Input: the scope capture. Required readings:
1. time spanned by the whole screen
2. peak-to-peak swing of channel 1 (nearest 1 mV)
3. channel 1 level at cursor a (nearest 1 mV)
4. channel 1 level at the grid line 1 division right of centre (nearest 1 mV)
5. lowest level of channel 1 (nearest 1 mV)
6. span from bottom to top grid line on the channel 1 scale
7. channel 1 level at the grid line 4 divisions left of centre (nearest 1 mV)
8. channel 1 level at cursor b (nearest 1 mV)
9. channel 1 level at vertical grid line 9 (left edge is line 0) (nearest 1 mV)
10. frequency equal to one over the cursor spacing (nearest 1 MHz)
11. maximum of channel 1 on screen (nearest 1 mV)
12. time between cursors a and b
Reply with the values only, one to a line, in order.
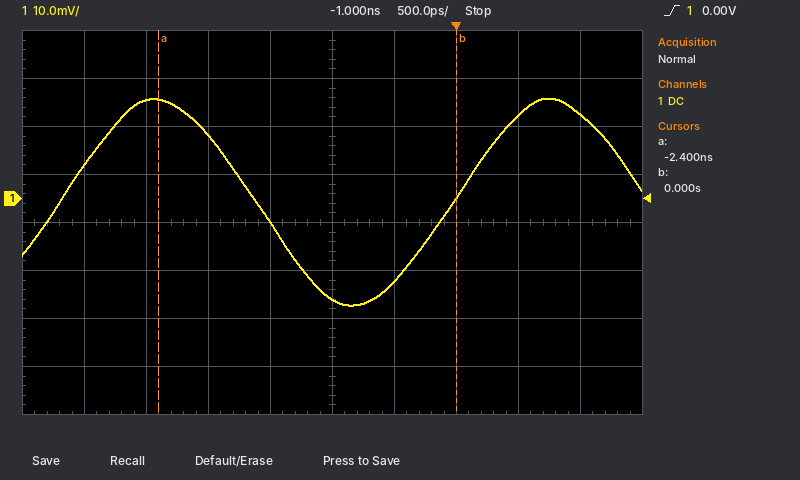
5 ns
43 mV
21 mV
-17 mV
-22 mV
80 mV
7 mV
0 mV
18 mV
417 MHz
21 mV
2.40 ns
